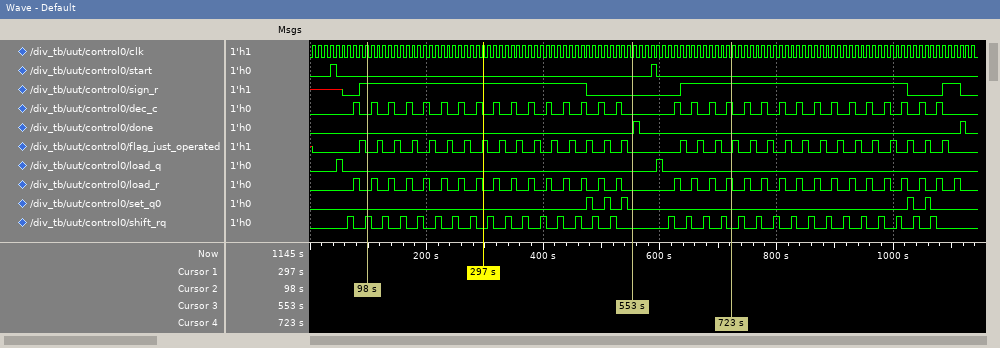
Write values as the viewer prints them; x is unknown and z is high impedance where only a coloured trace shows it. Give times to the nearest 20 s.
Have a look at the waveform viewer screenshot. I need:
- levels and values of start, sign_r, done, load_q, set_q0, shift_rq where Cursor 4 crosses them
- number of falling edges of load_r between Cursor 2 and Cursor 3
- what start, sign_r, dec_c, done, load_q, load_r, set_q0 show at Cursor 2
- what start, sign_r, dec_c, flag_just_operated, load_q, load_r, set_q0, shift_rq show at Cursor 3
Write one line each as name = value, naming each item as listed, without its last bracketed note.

levels and values of start, sign_r, done, load_q, set_q0, shift_rq where Cursor 4 crosses them = start=0, sign_r=1, done=0, load_q=0, set_q0=0, shift_rq=0
number of falling edges of load_r between Cursor 2 and Cursor 3 = 15
what start, sign_r, dec_c, done, load_q, load_r, set_q0 show at Cursor 2 = start=0, sign_r=1, dec_c=0, done=0, load_q=0, load_r=0, set_q0=0
what start, sign_r, dec_c, flag_just_operated, load_q, load_r, set_q0, shift_rq show at Cursor 3 = start=0, sign_r=0, dec_c=0, flag_just_operated=0, load_q=0, load_r=0, set_q0=0, shift_rq=0
